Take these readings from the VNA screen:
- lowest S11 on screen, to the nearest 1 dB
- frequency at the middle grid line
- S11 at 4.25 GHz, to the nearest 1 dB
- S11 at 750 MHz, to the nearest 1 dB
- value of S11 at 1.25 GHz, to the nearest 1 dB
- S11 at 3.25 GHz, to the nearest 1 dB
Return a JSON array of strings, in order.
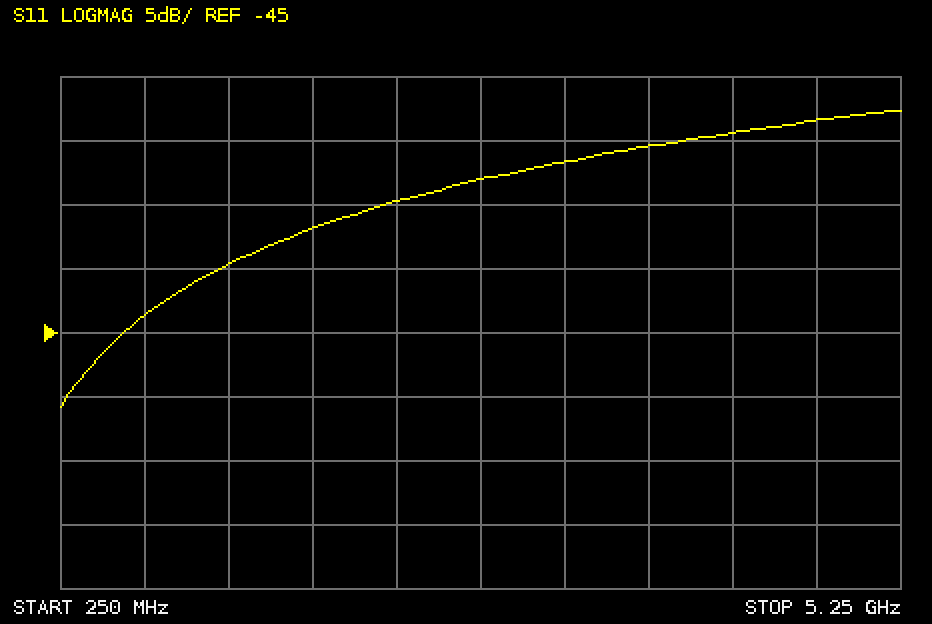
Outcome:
["-51 dB", "2.75 GHz", "-29 dB", "-44 dB", "-40 dB", "-32 dB"]
